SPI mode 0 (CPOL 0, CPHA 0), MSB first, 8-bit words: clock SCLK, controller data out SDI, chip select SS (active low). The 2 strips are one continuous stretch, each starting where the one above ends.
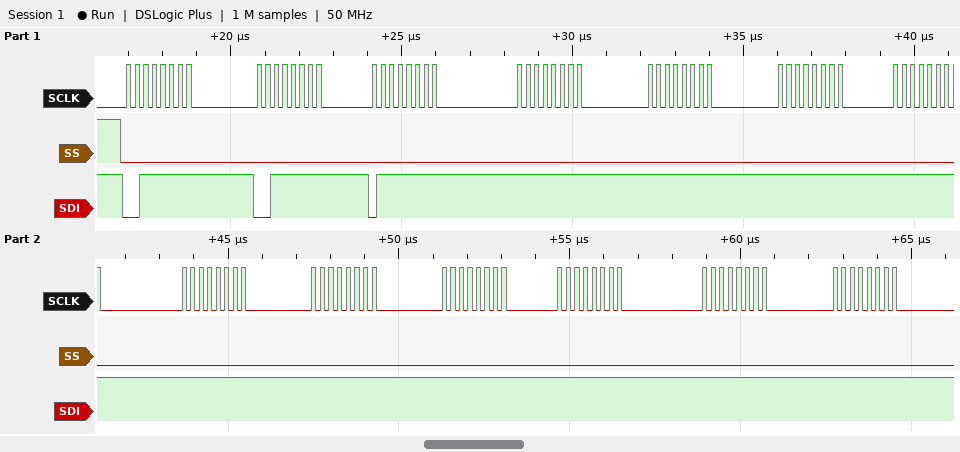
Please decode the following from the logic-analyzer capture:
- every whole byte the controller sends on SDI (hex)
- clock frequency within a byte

3F 3F 7F FF FF FF FF FF FF FF FF FF FF
4 MHz
